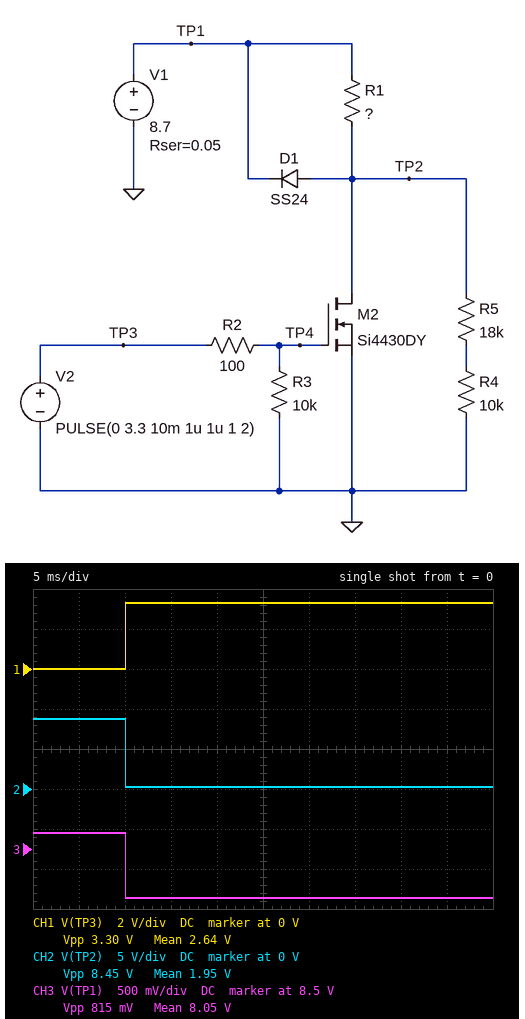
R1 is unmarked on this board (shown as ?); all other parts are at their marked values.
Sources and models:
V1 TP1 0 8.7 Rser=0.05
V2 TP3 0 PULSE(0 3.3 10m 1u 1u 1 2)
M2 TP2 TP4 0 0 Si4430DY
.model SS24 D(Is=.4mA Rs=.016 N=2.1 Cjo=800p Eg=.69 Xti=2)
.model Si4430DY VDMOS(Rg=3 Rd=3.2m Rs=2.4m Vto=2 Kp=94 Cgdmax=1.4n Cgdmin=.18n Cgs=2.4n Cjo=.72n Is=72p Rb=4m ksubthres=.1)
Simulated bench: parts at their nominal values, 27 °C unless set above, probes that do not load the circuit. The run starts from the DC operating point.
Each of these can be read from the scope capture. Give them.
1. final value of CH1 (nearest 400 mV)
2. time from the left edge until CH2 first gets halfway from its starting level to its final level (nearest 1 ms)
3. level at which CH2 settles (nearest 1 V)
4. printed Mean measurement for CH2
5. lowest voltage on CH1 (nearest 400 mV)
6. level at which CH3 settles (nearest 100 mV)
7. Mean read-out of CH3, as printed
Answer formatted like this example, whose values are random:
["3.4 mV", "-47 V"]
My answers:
["3.2 V", "10 ms", "0 V", "1.95 V", "0 V", "7.9 V", "8.05 V"]
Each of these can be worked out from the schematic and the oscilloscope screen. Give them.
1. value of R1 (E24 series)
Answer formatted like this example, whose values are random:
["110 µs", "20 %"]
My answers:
["0.47 Ω"]
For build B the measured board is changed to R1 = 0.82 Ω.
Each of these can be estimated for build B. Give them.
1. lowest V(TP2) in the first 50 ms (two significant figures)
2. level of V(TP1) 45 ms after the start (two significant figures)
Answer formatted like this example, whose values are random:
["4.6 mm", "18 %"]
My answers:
["140 mV", "8.2 V"]
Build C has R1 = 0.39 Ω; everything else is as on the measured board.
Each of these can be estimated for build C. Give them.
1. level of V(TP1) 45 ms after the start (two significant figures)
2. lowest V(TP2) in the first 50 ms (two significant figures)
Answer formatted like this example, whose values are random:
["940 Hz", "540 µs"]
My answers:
["7.7 V", "290 mV"]
